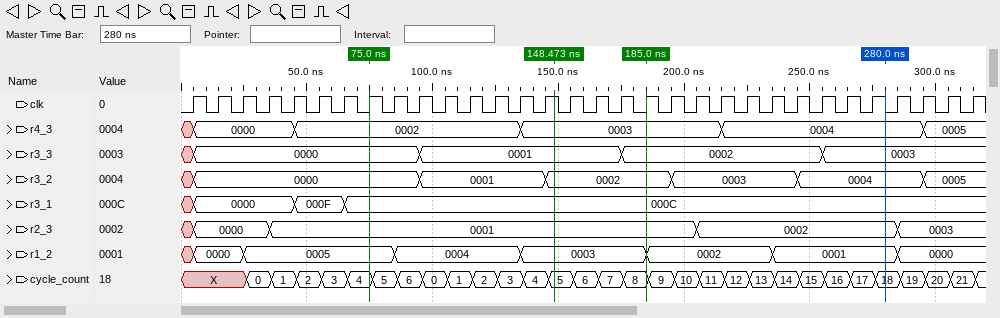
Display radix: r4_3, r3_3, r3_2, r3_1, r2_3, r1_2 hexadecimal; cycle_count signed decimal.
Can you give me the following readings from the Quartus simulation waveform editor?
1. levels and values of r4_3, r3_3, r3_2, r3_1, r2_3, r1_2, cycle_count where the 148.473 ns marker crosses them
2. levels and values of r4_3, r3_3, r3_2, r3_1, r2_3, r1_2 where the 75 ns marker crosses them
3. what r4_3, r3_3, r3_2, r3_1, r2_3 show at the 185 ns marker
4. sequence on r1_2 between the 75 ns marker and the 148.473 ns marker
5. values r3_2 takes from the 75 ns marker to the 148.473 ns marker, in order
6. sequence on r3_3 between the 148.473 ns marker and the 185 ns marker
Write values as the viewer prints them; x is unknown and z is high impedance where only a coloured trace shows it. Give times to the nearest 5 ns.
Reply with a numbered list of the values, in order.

1. r4_3=0003, r3_3=0001, r3_2=0002, r3_1=000C, r2_3=0001, r1_2=0003, cycle_count=5
2. r4_3=0002, r3_3=0000, r3_2=0000, r3_1=000C, r2_3=0001, r1_2=0005
3. r4_3=0003, r3_3=0002, r3_2=0002, r3_1=000C, r2_3=0001
4. 0005, 0004, 0003
5. 0000, 0001, 0002
6. 0001, 0002
